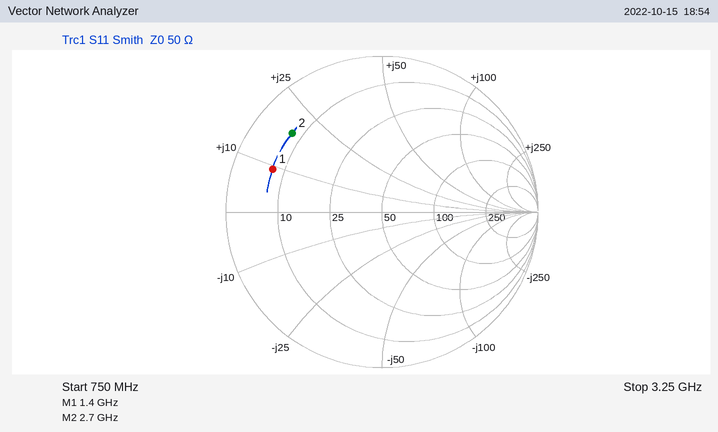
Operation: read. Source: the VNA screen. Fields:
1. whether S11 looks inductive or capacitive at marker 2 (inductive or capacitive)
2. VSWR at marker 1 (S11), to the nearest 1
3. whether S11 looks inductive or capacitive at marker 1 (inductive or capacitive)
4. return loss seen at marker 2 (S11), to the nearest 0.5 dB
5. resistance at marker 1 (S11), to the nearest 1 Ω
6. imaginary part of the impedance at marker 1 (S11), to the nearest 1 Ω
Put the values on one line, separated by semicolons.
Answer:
inductive; 7; inductive; 2.5 dB; 7 Ω; +9 Ω
